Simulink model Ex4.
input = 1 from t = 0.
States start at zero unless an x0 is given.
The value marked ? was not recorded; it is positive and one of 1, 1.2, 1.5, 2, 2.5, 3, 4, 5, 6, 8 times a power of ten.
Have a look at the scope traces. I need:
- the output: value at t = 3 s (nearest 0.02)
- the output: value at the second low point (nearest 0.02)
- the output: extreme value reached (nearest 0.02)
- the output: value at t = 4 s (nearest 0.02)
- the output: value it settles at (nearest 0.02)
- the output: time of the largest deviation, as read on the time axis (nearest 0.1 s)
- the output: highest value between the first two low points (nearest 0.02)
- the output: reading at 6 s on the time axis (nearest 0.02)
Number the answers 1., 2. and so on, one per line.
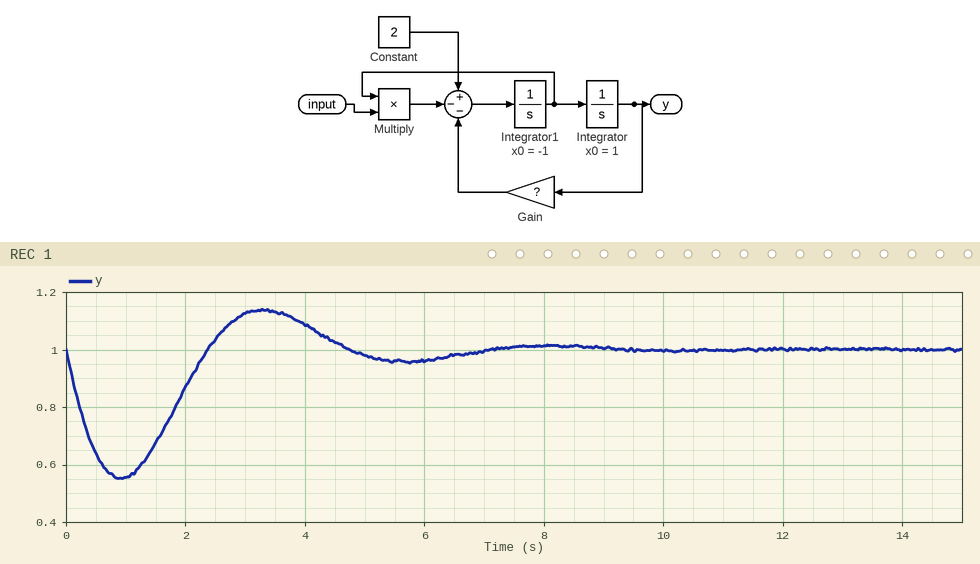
1. 1.12
2. 0.96
3. 0.56
4. 1.08
5. 1.00
6. 0.9 s
7. 1.14
8. 0.96
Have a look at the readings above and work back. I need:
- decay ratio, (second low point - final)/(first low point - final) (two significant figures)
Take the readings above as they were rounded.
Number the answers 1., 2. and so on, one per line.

1. 0.091
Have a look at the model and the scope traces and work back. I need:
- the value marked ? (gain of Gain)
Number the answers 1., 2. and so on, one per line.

1. 2
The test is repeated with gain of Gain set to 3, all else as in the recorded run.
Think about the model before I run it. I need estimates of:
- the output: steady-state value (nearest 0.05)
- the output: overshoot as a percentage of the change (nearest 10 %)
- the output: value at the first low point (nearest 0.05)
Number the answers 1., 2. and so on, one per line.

1. 0.65
2. 100 %
3. 0.35
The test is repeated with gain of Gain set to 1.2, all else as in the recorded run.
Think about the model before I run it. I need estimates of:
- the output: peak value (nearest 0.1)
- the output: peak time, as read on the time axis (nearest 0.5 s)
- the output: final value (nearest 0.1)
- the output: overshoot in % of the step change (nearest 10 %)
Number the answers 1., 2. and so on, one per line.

1. 1.9
2. 4.0 s
3. 1.7
4. 30 %
